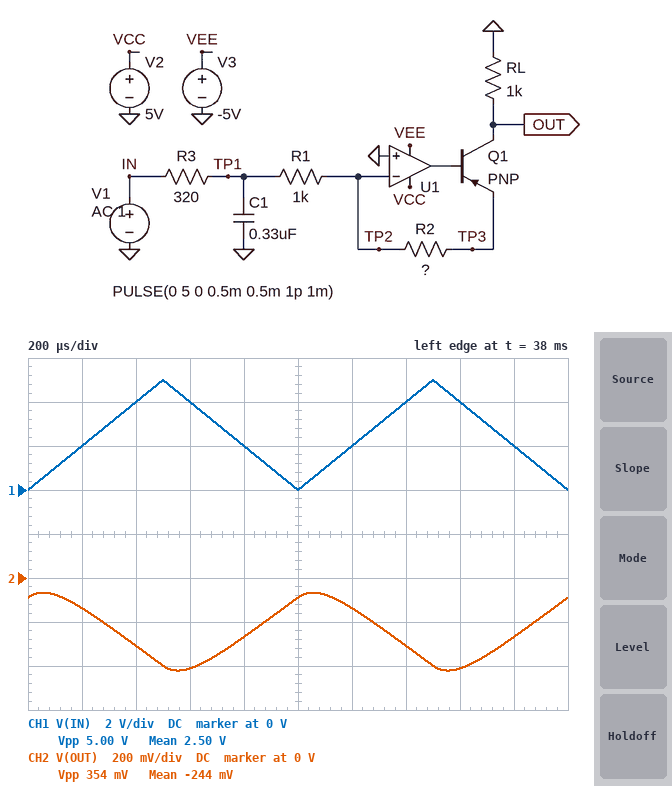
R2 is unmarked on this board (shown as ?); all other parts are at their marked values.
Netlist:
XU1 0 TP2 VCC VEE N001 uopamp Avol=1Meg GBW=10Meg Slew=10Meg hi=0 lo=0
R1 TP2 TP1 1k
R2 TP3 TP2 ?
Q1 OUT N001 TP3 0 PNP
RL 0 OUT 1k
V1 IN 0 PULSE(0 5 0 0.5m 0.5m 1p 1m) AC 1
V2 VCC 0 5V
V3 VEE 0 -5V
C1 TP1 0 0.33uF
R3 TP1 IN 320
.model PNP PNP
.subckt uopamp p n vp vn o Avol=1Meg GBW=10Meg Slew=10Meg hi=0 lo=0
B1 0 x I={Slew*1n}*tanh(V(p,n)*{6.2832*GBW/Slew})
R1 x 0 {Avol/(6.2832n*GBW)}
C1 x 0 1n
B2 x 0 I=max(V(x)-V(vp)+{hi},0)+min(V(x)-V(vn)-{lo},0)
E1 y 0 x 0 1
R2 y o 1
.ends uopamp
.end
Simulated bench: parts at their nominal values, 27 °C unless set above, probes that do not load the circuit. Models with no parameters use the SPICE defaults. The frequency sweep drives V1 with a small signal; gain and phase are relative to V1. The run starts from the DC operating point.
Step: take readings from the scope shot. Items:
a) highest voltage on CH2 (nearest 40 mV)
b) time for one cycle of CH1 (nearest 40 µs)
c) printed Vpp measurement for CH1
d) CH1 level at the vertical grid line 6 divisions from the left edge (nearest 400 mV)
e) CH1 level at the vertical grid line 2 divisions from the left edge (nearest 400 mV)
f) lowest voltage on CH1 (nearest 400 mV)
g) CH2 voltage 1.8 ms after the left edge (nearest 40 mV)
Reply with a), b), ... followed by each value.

a) -80 mV
b) 1.00 ms
c) 5.00 V
d) 2.0 V
e) 4.0 V
f) 0 V
g) -280 mV
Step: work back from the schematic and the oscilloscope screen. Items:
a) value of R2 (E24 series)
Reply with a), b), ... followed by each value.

a) 120 Ω
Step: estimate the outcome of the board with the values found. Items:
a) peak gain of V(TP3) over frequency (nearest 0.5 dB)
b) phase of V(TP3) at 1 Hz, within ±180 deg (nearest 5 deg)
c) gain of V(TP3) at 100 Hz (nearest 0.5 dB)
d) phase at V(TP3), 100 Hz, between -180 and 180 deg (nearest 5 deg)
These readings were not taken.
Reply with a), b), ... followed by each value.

a) 0 dB
b) 0 deg
c) 0 dB
d) -5 deg
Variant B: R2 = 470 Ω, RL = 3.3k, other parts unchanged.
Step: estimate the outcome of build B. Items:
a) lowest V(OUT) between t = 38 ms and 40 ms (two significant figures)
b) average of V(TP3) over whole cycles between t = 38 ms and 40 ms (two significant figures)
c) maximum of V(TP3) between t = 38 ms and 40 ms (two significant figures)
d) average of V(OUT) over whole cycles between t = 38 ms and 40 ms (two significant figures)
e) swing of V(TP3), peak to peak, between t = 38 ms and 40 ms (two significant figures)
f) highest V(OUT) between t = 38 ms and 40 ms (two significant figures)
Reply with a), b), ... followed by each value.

a) -1.6 V
b) -890 mV
c) -200 mV
d) -910 mV
e) 1.4 V
f) -210 mV
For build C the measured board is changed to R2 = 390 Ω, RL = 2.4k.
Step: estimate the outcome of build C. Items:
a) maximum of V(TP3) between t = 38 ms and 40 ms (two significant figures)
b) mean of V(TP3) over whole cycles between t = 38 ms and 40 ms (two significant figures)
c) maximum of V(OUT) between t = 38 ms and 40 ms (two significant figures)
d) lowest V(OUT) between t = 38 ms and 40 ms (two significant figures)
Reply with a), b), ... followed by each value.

a) -160 mV
b) -740 mV
c) -180 mV
d) -1.3 V
